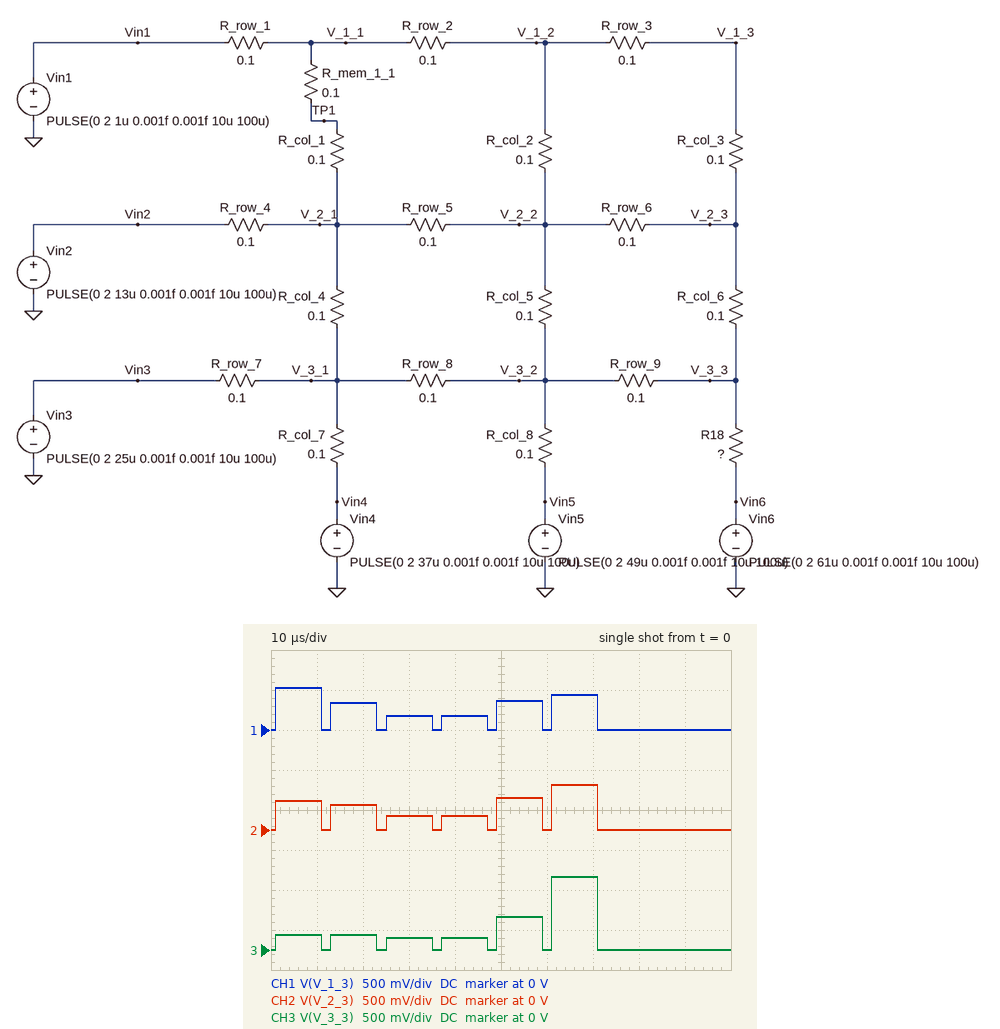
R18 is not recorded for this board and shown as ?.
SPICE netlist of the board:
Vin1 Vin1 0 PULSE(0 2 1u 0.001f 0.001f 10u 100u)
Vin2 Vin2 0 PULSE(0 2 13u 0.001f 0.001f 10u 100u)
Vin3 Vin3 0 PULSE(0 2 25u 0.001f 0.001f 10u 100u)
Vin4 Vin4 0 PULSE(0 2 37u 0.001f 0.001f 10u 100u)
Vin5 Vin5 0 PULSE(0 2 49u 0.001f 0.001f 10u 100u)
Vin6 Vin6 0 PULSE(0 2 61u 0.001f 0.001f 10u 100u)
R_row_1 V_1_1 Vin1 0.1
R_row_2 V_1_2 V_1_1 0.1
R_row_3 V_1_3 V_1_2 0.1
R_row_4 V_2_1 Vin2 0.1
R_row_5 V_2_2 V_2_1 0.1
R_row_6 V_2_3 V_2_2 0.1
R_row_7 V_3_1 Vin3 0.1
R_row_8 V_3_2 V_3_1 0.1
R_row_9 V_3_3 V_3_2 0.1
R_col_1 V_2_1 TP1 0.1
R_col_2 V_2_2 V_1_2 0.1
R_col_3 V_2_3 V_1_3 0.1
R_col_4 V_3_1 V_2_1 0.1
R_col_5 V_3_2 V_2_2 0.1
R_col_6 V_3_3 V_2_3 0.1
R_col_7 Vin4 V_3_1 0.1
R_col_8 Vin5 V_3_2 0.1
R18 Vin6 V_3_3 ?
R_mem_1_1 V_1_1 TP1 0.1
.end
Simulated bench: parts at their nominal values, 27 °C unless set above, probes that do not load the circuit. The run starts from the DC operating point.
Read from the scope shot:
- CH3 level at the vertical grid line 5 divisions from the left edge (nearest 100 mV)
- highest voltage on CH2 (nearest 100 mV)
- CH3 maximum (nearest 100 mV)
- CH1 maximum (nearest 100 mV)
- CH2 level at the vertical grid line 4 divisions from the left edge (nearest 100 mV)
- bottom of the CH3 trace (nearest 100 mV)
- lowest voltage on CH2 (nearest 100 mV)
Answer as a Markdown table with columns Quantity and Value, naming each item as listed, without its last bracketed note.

| Quantity | Value |
|---|---|
| CH3 level at the vertical grid line 5 divisions from the left edge | 400 mV |
| highest voltage on CH2 | 600 mV |
| CH3 maximum | 900 mV |
| CH1 maximum | 500 mV |
| CH2 level at the vertical grid line 4 divisions from the left edge | 200 mV |
| bottom of the CH3 trace | 0 V |
| lowest voltage on CH2 | 0 V |
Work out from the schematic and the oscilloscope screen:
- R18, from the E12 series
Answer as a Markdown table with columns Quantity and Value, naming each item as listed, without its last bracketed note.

| Quantity | Value |
|---|---|
| R18, from the E12 series | 0.12 Ω |
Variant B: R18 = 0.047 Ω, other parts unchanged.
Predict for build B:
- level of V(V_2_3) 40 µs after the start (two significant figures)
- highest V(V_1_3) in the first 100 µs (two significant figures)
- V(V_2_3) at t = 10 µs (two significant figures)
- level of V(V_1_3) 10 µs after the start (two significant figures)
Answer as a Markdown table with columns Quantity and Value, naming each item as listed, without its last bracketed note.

| Quantity | Value |
|---|---|
| level of V(V_2_3) 40 µs after the start | 140 mV |
| highest V(V_1_3) in the first 100 µs | 660 mV |
| V(V_2_3) at t = 10 µs | 310 mV |
| level of V(V_1_3) 10 µs after the start | 480 mV |
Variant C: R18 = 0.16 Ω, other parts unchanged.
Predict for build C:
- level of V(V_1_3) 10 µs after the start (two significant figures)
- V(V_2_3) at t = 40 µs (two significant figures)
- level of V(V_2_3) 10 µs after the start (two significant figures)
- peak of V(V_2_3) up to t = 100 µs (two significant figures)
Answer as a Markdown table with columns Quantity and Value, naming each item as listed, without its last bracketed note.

| Quantity | Value |
|---|---|
| level of V(V_1_3) 10 µs after the start | 530 mV |
| V(V_2_3) at t = 40 µs | 190 mV |
| level of V(V_2_3) 10 µs after the start | 380 mV |
| peak of V(V_2_3) up to t = 100 µs | 480 mV |
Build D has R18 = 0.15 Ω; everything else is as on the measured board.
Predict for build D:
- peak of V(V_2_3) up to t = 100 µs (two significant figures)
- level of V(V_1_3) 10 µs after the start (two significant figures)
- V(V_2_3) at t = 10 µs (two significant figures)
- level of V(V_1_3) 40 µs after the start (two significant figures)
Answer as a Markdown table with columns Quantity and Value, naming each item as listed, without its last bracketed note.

| Quantity | Value |
|---|---|
| peak of V(V_2_3) up to t = 100 µs | 500 mV |
| level of V(V_1_3) 10 µs after the start | 530 mV |
| V(V_2_3) at t = 10 µs | 370 mV |
| level of V(V_1_3) 40 µs after the start | 180 mV |
